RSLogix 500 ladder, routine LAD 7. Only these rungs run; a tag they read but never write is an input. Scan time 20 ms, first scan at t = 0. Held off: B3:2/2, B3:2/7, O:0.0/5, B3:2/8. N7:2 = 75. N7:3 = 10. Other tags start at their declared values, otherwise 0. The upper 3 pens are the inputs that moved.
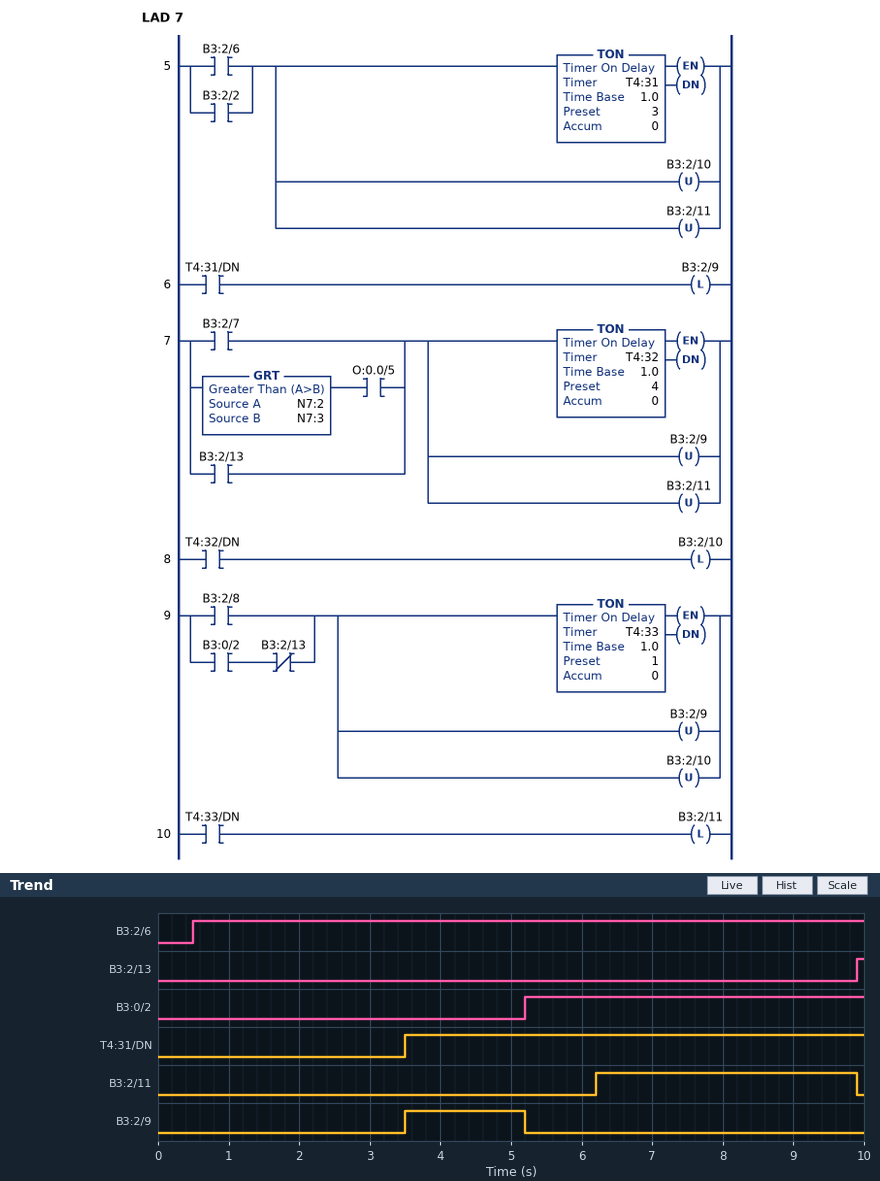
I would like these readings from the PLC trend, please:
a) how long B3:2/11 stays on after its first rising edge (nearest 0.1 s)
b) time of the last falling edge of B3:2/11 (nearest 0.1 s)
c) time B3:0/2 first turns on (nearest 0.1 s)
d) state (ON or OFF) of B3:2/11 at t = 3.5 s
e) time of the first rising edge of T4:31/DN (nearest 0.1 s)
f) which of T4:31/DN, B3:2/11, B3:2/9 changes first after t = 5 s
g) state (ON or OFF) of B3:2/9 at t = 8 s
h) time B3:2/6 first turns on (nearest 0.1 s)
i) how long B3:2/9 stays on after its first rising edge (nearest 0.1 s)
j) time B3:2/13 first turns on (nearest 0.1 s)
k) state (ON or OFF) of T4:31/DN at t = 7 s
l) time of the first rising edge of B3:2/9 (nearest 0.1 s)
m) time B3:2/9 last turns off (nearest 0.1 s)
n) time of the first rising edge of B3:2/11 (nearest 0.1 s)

3.7 s
9.9 s
5.2 s
OFF
3.5 s
B3:2/9
OFF
0.5 s
1.7 s
9.9 s
ON
3.5 s
5.2 s
6.2 s
